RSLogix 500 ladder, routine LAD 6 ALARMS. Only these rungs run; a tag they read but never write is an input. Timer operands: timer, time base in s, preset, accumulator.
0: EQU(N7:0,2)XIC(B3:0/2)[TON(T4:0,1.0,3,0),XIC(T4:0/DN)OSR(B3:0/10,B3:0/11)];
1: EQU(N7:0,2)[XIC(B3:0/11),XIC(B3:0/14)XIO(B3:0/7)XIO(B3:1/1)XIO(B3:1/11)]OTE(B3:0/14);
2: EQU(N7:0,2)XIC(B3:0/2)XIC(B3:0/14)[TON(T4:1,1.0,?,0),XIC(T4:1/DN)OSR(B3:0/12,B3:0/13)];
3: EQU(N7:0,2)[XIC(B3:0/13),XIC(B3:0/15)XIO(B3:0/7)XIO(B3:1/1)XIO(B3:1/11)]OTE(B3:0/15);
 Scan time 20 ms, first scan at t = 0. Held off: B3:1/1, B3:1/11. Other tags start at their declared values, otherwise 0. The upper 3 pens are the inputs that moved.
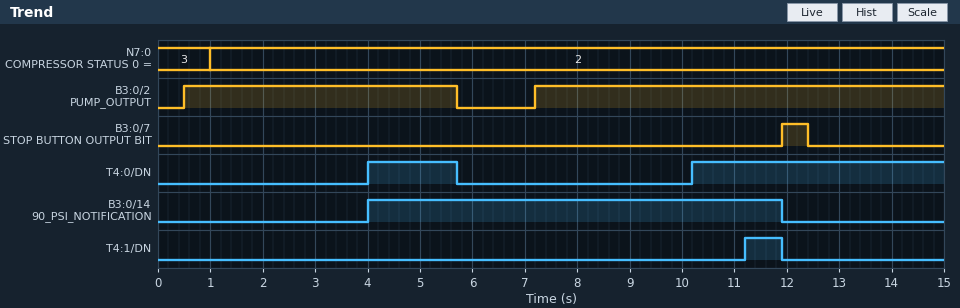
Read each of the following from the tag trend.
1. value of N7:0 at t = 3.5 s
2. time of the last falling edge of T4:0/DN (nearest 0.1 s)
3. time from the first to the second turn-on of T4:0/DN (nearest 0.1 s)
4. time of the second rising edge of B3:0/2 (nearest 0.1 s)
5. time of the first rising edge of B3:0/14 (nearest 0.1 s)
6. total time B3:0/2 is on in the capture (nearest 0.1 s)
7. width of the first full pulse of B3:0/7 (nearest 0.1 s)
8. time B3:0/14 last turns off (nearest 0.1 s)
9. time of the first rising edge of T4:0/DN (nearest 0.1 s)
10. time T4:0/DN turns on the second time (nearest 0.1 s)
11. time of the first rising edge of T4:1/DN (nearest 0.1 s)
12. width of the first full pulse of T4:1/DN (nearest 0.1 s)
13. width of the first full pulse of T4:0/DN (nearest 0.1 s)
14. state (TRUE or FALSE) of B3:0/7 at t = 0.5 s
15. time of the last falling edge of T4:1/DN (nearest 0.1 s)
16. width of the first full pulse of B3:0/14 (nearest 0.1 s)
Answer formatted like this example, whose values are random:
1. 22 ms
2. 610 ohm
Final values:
1. 2
2. 5.7 s
3. 6.2 s
4. 7.2 s
5. 4.0 s
6. 13.0 s
7. 0.5 s
8. 11.9 s
9. 4.0 s
10. 10.2 s
11. 11.2 s
12. 0.7 s
13. 1.7 s
14. FALSE
15. 11.9 s
16. 7.9 s
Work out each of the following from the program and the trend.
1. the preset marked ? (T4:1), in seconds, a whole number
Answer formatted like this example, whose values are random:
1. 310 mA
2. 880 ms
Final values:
1. 4 s
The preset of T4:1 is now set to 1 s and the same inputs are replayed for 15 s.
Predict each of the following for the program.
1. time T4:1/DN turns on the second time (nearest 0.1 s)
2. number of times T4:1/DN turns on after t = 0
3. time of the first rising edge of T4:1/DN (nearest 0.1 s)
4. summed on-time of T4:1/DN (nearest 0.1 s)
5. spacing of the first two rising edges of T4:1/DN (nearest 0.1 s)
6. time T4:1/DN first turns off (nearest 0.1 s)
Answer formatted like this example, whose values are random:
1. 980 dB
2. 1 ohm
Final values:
1. 8.2 s
2. 2
3. 5.0 s
4. 4.4 s
5. 3.2 s
6. 5.7 s
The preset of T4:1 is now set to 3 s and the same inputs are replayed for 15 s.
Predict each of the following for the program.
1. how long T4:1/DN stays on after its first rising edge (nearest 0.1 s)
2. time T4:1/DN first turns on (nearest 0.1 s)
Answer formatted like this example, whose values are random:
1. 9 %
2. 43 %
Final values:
1. 1.7 s
2. 10.2 s
